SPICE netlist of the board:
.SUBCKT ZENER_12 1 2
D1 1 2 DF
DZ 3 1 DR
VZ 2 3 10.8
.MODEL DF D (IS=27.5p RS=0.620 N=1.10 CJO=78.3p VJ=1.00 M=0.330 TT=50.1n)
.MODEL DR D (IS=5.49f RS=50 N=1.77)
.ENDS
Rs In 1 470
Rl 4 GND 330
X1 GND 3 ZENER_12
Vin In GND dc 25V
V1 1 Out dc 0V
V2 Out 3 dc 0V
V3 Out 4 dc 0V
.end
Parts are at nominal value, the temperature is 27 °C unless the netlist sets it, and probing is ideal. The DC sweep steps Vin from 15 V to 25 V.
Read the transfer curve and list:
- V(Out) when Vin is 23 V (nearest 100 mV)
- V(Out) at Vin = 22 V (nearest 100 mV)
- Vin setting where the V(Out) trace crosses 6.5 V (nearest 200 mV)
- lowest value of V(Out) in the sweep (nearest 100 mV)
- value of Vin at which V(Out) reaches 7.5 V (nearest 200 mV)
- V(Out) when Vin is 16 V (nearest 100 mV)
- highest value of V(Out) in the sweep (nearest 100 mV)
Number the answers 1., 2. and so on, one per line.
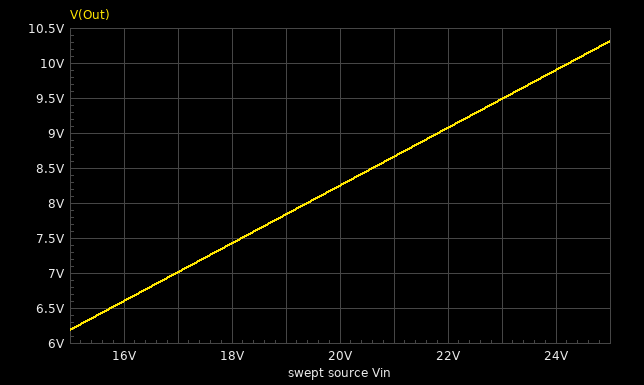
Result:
1. 9.5 V
2. 9.1 V
3. 15.8 V
4. 6.2 V
5. 18.2 V
6. 6.6 V
7. 10.3 V
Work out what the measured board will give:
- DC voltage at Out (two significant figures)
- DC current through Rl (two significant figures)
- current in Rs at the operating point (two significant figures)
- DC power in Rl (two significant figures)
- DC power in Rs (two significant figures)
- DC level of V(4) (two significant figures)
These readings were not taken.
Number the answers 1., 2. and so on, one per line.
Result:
1. 10 V
2. 31 mA
3. 31 mA
4. 320 mW
5. 460 mW
6. 10 V
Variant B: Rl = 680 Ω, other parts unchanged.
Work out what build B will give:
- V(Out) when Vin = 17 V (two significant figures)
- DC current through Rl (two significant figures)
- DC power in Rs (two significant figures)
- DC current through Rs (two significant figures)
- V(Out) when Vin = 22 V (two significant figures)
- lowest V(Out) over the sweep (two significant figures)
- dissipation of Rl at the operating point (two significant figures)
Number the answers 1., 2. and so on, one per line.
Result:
1. 10 V
2. 18 mA
3. 330 mW
4. 27 mA
5. 12 V
6. 8.9 V
7. 230 mW
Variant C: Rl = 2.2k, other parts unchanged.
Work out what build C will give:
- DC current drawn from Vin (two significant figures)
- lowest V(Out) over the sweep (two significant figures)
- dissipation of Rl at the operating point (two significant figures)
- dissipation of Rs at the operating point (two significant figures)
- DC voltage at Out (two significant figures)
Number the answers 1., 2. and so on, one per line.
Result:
1. 25 mA
2. 12 V
3. 78 mW
4. 300 mW
5. 13 V
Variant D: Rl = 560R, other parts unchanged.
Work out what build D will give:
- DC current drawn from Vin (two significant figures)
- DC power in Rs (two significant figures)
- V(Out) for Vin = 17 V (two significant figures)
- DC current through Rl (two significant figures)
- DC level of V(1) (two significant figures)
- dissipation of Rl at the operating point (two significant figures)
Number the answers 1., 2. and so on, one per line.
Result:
1. 27 mA
2. 340 mW
3. 9.2 V
4. 22 mA
5. 12 V
6. 270 mW
